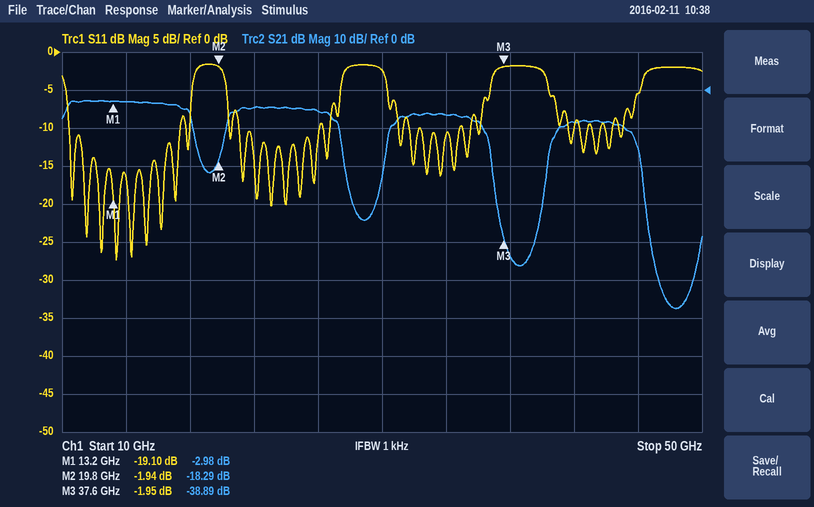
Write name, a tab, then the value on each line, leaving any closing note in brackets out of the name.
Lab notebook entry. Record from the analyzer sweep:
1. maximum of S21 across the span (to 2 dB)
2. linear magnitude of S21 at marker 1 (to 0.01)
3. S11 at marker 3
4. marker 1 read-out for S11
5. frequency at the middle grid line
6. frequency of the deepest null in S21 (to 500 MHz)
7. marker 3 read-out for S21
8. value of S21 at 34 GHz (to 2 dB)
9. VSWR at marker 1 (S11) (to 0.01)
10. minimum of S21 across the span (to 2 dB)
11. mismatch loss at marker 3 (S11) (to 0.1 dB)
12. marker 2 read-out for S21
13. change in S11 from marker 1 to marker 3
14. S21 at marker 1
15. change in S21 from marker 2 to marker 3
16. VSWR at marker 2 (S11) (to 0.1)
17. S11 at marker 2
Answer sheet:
maximum of S21 across the span	-2 dB
linear magnitude of S21 at marker 1	0.71
S11 at marker 3	-1.95 dB
marker 1 read-out for S11	-19.10 dB
frequency at the middle grid line	30 GHz
frequency of the deepest null in S21	48.5 GHz
marker 3 read-out for S21	-38.89 dB
value of S21 at 34 GHz	-6 dB
VSWR at marker 1 (S11)	1.25
minimum of S21 across the span	-58 dB
mismatch loss at marker 3 (S11)	4.4 dB
marker 2 read-out for S21	-18.29 dB
change in S11 from marker 1 to marker 3	17.15 dB
S21 at marker 1	-2.98 dB
change in S21 from marker 2 to marker 3	-20.60 dB
VSWR at marker 2 (S11)	9.0
S11 at marker 2	-1.94 dB
